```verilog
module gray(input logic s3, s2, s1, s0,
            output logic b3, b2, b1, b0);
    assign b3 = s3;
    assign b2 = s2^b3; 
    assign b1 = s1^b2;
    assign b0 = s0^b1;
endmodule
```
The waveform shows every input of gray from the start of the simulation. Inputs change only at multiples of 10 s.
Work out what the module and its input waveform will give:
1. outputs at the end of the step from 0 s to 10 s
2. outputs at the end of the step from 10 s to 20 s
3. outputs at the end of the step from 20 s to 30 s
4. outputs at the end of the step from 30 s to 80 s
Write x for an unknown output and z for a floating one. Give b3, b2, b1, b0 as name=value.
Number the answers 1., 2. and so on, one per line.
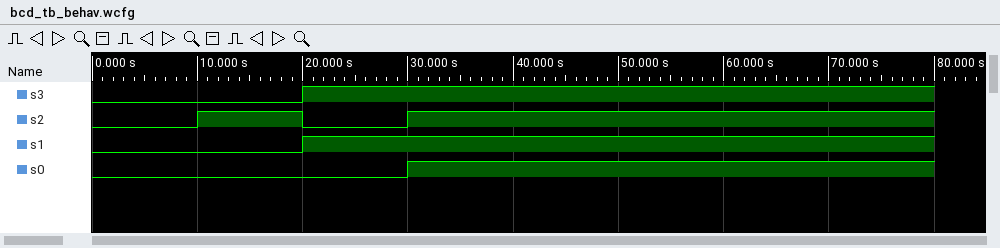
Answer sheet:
1. b3=0, b2=0, b1=0, b0=0
2. b3=0, b2=1, b1=1, b0=1
3. b3=1, b2=1, b1=0, b0=0
4. b3=1, b2=0, b1=1, b0=0
